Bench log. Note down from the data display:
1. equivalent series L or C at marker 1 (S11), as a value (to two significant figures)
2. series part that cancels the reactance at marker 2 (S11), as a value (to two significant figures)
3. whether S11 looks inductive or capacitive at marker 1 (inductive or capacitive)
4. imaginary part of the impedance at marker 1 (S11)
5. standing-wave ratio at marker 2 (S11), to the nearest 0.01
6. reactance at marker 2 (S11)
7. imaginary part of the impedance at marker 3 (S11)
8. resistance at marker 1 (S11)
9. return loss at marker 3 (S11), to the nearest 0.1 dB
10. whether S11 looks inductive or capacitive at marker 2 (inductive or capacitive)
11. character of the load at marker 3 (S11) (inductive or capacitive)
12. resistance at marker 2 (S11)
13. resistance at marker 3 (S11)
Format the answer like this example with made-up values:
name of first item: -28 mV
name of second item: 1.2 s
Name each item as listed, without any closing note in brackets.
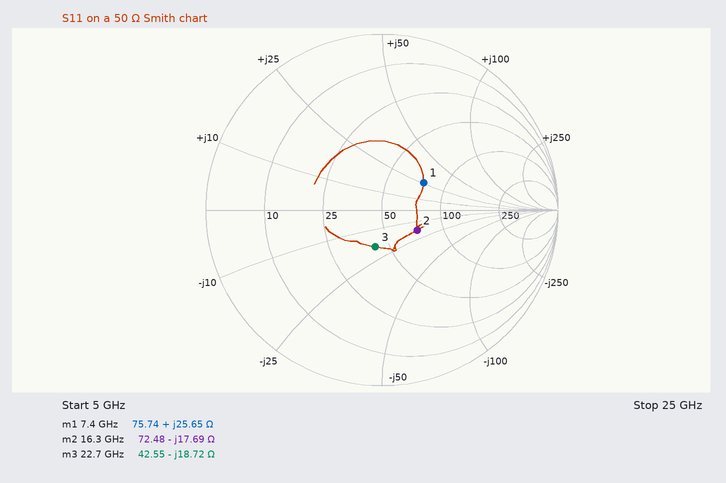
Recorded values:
equivalent series L or C at marker 1 (S11), as a value: 550 pH
series part that cancels the reactance at marker 2 (S11), as a value: 170 pH
whether S11 looks inductive or capacitive at marker 1: inductive
imaginary part of the impedance at marker 1: +25.65 Ω
standing-wave ratio at marker 2 (S11), to the nearest 0.01: 1.60
reactance at marker 2: -17.69 Ω
imaginary part of the impedance at marker 3: -18.72 Ω
resistance at marker 1: 75.74 Ω
return loss at marker 3 (S11), to the nearest 0.1 dB: 13.4 dB
whether S11 looks inductive or capacitive at marker 2: capacitive
character of the load at marker 3 (S11): capacitive
resistance at marker 2: 72.48 Ω
resistance at marker 3: 42.55 Ω
